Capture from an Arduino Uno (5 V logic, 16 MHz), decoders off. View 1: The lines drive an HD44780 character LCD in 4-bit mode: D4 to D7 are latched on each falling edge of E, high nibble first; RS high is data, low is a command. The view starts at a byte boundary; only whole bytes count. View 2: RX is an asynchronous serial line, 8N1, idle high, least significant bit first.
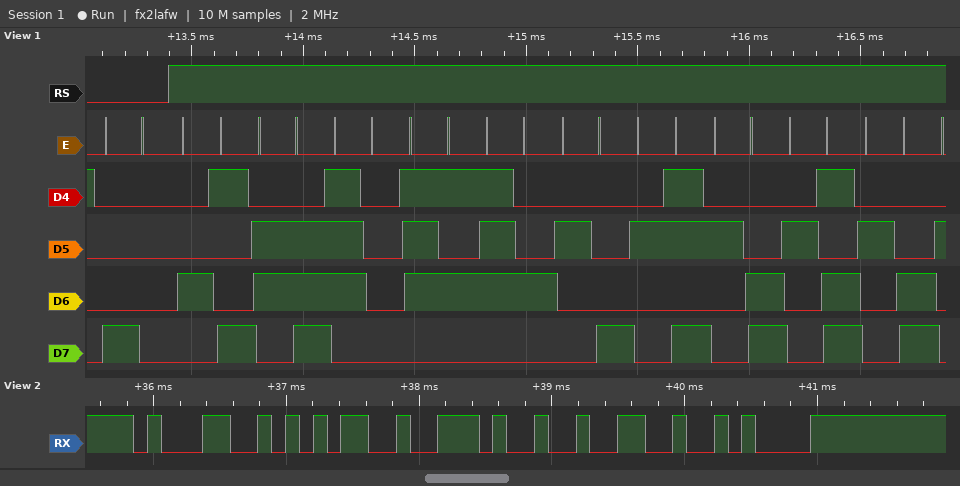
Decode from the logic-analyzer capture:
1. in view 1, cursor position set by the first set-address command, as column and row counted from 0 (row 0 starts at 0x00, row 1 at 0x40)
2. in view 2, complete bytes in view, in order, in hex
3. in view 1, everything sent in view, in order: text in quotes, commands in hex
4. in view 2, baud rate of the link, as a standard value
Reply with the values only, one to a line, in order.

column 0, row 0
0x31 0x35 0x2E 0x32 0x0A
0x80 "Input(+,-,"
9600 baud
